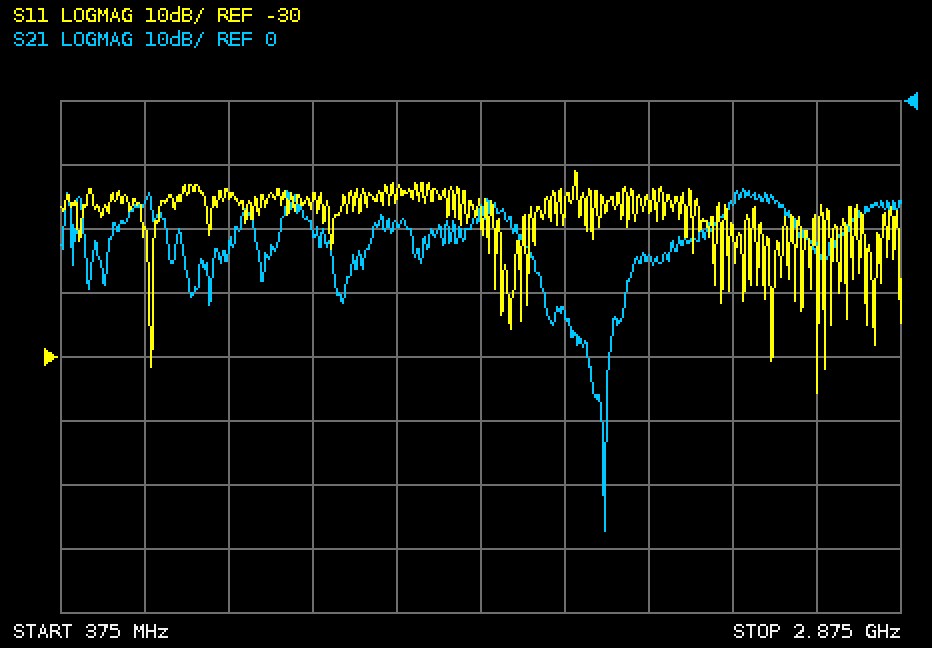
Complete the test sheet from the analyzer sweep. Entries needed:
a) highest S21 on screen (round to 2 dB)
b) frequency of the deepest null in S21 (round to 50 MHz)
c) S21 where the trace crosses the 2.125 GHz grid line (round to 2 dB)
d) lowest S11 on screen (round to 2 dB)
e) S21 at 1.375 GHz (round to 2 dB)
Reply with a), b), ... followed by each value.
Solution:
a) -14 dB
b) 2.00 GHz
c) -24 dB
d) -36 dB
e) -20 dB
